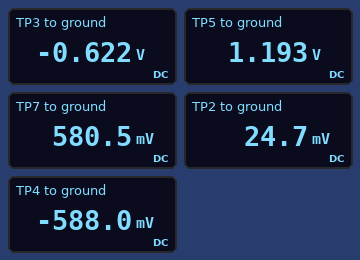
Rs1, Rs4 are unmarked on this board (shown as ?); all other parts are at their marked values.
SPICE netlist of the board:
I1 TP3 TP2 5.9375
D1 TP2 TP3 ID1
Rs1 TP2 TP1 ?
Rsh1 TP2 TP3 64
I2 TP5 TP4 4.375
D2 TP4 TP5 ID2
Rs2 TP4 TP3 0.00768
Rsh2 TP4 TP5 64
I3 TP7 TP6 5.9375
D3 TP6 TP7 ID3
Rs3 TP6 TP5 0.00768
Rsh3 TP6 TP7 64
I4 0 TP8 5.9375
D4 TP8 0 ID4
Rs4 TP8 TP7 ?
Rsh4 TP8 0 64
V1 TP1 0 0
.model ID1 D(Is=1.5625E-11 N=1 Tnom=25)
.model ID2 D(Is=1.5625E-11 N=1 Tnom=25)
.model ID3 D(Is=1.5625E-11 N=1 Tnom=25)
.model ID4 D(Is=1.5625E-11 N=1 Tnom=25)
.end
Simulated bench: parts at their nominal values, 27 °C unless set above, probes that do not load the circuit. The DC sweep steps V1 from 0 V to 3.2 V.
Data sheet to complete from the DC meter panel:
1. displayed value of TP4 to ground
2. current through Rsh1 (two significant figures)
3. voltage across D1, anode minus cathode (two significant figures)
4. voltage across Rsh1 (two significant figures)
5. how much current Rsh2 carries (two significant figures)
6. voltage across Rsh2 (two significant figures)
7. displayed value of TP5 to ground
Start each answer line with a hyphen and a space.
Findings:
- -588.0 mV
- 10 mA
- 650 mV
- 650 mV
- 28 mA
- 1.8 V
- 1.193 V
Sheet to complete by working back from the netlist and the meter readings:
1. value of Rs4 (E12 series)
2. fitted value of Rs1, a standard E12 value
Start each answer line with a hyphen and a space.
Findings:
- 0.015 Ω
- 5.6 mΩ
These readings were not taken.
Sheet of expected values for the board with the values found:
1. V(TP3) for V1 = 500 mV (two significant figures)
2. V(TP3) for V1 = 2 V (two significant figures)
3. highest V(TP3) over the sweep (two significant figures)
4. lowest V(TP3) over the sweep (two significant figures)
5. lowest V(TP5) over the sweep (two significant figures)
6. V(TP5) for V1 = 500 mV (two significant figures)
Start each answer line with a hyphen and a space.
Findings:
- -120 mV
- 1.4 V
- 2.4 V
- -620 mV
- 1.2 V
- 1.2 V
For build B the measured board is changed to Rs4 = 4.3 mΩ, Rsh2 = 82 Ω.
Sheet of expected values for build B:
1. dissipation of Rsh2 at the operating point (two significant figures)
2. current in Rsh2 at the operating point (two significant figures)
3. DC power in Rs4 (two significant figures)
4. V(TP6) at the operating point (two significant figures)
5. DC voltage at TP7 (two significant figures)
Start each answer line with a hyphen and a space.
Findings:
- 41 mW
- 22 mA
- 83 mW
- 1.3 V
- 630 mV
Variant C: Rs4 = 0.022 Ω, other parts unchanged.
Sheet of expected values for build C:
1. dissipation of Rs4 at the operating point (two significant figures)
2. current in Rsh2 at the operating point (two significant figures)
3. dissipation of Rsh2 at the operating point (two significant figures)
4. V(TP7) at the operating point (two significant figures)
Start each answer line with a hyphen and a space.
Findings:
- 430 mW
- 27 mA
- 48 mW
- 550 mV
